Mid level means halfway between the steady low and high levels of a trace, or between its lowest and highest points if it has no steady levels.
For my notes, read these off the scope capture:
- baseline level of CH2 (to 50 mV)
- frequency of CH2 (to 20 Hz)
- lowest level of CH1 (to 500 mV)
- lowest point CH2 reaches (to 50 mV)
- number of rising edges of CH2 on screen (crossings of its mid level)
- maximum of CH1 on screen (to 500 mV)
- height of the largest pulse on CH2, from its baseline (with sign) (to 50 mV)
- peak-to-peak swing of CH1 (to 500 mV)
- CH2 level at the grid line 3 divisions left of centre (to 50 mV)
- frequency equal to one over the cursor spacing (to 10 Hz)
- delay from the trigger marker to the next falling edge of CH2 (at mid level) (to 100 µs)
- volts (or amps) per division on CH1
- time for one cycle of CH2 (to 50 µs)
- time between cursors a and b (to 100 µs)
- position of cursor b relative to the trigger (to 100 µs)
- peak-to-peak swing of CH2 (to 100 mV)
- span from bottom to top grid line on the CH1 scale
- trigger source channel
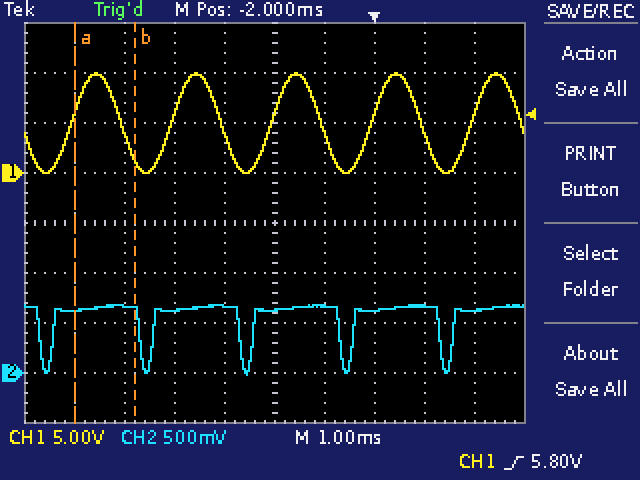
650 mV
500 Hz
0.0 V
0 mV
5
10.0 V
-650 mV
10.0 V
650 mV
830 Hz
1.3 ms
5 V
2.00 ms
1.2 ms
-4.8 ms
700 mV
40 V
CH1
